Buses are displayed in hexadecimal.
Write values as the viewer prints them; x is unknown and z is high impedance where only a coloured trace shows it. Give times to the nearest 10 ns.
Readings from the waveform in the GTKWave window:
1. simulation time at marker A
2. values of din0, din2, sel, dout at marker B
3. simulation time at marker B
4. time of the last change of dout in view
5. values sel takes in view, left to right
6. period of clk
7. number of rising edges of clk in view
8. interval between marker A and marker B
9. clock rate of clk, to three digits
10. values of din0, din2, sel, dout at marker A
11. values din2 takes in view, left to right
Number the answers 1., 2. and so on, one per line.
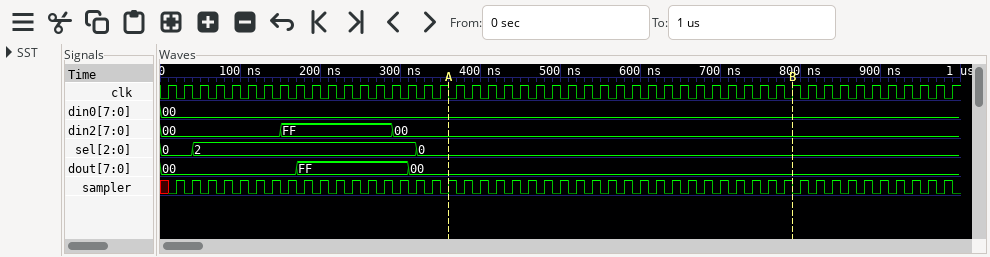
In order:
1. 360 ns
2. din0=00, din2=00, sel=0, dout=00
3. 790 ns
4. 310 ns
5. 0, 2, 0
6. 20 ns
7. 50
8. 430 ns
9. 50.0 MHz
10. din0=00, din2=00, sel=0, dout=00
11. 00, FF, 00
